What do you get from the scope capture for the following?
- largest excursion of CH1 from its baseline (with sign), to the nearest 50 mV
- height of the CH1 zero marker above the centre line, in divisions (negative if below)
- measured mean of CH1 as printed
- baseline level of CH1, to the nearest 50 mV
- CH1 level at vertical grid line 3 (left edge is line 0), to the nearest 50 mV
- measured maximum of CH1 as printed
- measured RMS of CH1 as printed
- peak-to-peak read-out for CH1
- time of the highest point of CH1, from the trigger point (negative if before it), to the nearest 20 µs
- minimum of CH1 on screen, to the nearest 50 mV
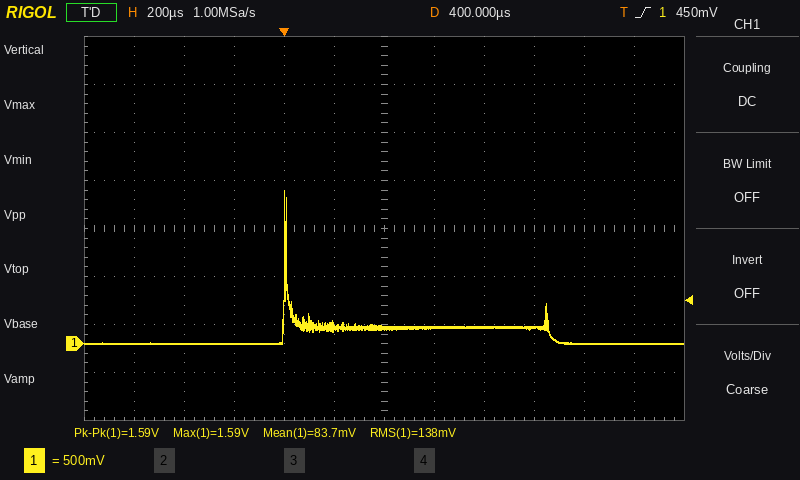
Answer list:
+1.60 V
-2.4 div
83.7 mV
0 mV
0 mV
1.59 V
138 mV
1.59 V
0 µs
0 mV
